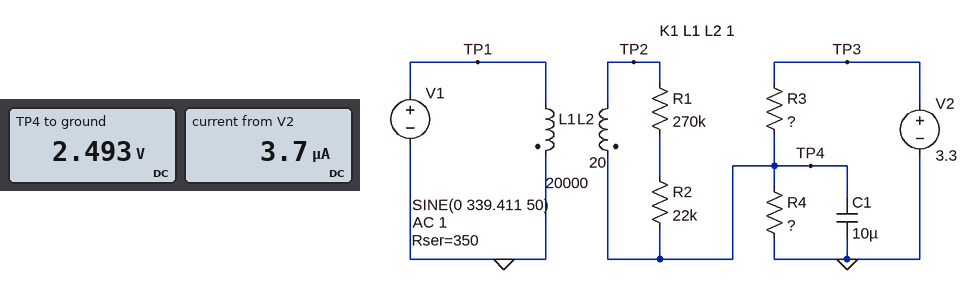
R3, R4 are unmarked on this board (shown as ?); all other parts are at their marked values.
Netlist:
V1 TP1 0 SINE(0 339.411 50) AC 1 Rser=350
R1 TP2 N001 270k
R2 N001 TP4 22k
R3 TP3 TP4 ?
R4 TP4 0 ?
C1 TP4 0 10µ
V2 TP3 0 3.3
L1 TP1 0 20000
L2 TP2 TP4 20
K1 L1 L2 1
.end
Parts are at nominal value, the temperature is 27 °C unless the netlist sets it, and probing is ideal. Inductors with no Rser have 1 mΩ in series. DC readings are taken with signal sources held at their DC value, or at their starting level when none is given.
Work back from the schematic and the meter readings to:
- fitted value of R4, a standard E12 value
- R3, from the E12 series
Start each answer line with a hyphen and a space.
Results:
- 680 kΩ
- 220 kΩ
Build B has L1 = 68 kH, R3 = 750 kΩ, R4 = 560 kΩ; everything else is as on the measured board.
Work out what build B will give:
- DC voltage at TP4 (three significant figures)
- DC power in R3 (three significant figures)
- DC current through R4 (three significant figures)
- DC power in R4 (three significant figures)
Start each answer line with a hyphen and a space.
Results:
- 1.41 V
- 4.76 µW
- 2.52 µA
- 3.55 µW
